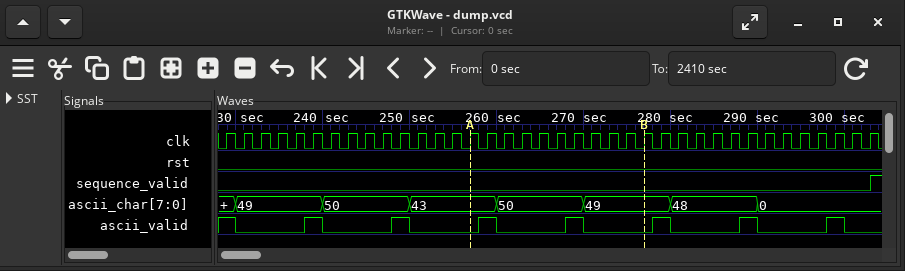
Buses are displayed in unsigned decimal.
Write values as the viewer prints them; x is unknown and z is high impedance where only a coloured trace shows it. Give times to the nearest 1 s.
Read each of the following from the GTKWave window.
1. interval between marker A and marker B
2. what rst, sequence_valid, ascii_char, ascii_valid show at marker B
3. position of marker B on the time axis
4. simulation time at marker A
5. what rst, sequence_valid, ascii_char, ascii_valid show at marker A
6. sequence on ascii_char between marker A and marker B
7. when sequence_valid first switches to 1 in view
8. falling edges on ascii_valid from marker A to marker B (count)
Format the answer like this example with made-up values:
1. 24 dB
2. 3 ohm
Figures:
1. 20 s
2. rst=0, sequence_valid=0, ascii_char=49, ascii_valid=0
3. 277 s
4. 257 s
5. rst=0, sequence_valid=0, ascii_char=43, ascii_valid=0
6. 43, 50, 49
7. 303 s
8. 2
